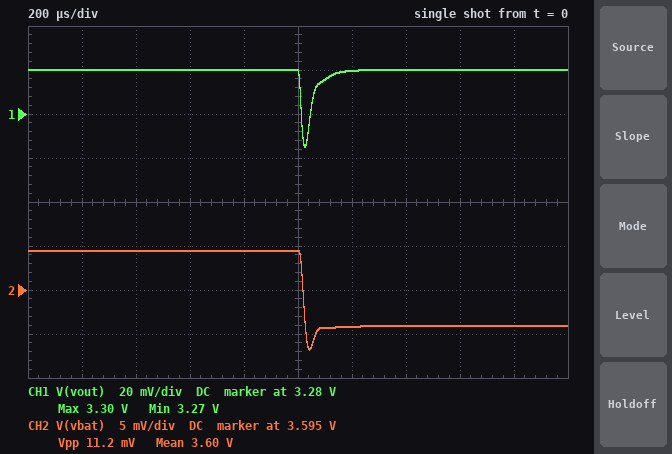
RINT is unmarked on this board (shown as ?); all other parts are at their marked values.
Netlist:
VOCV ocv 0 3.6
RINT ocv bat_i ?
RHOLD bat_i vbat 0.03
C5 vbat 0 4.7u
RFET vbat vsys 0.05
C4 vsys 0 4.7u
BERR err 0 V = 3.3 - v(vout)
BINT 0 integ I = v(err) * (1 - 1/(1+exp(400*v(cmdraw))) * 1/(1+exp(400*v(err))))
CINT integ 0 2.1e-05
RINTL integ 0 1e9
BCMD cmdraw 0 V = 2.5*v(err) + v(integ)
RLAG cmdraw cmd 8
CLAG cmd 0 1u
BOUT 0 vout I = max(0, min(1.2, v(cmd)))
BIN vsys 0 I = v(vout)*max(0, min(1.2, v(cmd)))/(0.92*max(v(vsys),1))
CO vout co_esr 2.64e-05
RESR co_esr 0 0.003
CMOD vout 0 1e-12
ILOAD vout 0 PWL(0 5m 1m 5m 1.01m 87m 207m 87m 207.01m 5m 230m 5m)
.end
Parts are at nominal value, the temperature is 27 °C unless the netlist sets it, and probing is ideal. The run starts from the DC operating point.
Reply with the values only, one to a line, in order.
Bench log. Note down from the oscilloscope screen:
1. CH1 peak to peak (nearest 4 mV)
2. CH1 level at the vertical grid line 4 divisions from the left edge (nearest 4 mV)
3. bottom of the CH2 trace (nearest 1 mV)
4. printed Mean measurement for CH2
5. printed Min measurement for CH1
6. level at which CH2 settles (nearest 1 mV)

36 mV
3.300 V
3.588 V
3.60 V
3.27 V
3.591 V
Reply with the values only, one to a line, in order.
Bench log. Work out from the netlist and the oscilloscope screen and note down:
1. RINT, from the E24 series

0.075 Ω
